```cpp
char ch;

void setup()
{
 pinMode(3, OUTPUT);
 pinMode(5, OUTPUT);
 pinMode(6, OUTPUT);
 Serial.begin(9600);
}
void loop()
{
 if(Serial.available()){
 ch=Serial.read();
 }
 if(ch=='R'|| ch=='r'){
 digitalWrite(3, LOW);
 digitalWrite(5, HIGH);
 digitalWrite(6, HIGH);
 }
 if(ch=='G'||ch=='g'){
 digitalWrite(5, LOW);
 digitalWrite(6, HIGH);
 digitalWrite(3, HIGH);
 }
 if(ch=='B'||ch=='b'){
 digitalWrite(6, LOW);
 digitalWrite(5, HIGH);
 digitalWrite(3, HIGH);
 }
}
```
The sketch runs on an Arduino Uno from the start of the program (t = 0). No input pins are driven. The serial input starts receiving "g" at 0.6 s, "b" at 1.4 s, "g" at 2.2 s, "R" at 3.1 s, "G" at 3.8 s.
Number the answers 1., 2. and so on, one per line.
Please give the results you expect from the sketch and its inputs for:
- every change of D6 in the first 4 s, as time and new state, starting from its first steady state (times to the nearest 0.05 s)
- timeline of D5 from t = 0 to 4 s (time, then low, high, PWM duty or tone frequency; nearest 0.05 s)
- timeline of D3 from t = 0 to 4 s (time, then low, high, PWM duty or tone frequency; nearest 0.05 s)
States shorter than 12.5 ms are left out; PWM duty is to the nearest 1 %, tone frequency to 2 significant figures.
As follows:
1. 0 s low; 0.6 s high; 1.4 s low; 2.2 s high
2. 0 s low; 1.4 s high; 2.2 s low; 3.1 s high; 3.8 s low
3. 0 s low; 0.6 s high; 3.1 s low; 3.8 s high
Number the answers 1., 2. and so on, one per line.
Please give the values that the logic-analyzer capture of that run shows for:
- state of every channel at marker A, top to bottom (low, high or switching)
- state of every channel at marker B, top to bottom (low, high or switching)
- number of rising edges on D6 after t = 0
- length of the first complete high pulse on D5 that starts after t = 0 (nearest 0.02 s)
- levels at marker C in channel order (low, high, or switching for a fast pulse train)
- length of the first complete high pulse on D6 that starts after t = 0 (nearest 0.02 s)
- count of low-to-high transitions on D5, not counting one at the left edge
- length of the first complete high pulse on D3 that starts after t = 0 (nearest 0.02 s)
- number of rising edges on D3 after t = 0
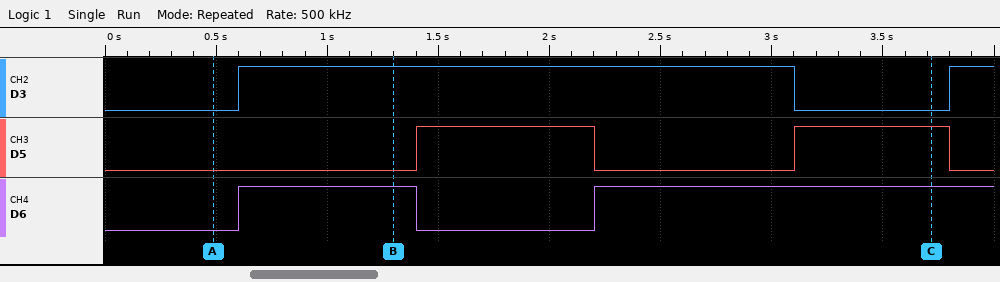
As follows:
1. D3 low, D5 low, D6 low
2. D3 high, D5 low, D6 high
3. 2
4. 0.80 s
5. D3 low, D5 high, D6 high
6. 0.80 s
7. 2
8. 2.50 s
9. 2
